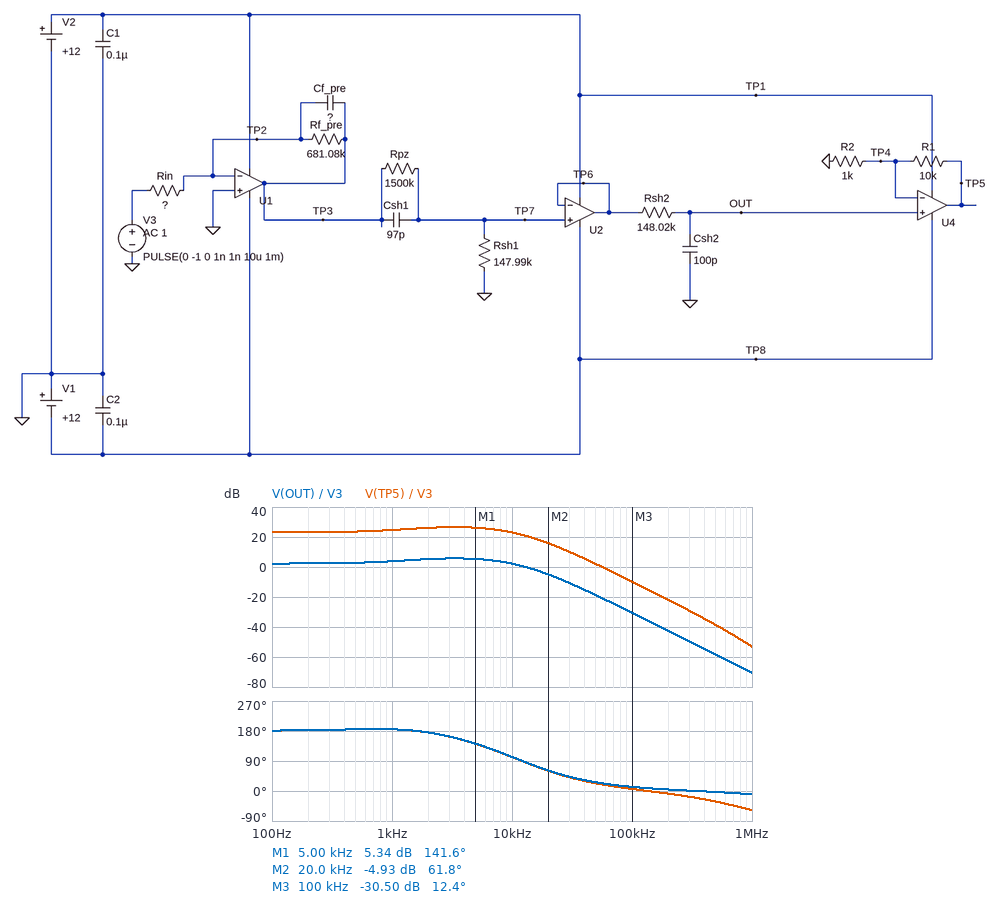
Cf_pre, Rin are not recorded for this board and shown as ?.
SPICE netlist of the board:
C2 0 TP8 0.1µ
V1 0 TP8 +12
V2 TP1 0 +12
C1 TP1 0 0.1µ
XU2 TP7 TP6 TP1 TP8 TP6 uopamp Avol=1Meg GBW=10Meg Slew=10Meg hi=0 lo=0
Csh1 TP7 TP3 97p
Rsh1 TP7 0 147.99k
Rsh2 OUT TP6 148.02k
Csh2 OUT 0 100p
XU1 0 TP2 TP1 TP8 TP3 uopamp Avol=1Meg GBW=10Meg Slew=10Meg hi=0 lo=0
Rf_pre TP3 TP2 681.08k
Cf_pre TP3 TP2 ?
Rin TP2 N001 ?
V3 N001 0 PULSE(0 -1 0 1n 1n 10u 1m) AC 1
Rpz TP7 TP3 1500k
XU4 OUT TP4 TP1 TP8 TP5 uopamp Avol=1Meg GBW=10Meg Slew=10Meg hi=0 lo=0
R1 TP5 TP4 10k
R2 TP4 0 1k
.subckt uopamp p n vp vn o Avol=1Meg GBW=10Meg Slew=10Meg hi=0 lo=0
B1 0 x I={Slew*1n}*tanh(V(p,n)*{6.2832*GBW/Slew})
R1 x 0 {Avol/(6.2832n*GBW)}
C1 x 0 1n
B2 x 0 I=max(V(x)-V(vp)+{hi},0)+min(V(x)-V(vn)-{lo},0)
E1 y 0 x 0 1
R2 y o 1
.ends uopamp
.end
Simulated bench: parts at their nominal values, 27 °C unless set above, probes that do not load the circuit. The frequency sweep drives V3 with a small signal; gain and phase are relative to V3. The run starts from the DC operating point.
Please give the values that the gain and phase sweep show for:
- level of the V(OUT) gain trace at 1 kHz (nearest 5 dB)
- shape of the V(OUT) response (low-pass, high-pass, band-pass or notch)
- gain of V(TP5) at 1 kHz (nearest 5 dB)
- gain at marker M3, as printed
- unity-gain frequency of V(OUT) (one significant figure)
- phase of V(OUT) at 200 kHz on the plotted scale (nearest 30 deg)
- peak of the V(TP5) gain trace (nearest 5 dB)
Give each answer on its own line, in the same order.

5 dB
low-pass
25 dB
-30.50 dB
10 kHz
0 deg
25 dB
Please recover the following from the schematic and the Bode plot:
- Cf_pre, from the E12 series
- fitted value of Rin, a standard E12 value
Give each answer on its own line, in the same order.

120 pF
47 kΩ
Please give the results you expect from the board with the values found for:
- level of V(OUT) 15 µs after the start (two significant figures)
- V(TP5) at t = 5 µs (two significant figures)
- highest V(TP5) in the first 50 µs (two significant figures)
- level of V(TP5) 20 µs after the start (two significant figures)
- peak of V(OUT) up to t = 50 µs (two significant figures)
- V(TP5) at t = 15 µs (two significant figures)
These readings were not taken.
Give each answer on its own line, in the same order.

540 mV
1.2 V
6.2 V
6.2 V
570 mV
5.9 V
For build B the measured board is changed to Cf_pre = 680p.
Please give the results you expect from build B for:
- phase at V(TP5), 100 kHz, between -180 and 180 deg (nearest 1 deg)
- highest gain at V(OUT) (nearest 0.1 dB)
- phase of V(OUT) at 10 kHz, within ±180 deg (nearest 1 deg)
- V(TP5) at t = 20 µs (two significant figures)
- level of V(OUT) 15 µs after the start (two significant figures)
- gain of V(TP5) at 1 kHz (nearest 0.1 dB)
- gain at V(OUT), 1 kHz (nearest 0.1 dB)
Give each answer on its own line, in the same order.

5 deg
2.3 dB
93 deg
1.2 V
100 mV
15.9 dB
-4.9 dB
